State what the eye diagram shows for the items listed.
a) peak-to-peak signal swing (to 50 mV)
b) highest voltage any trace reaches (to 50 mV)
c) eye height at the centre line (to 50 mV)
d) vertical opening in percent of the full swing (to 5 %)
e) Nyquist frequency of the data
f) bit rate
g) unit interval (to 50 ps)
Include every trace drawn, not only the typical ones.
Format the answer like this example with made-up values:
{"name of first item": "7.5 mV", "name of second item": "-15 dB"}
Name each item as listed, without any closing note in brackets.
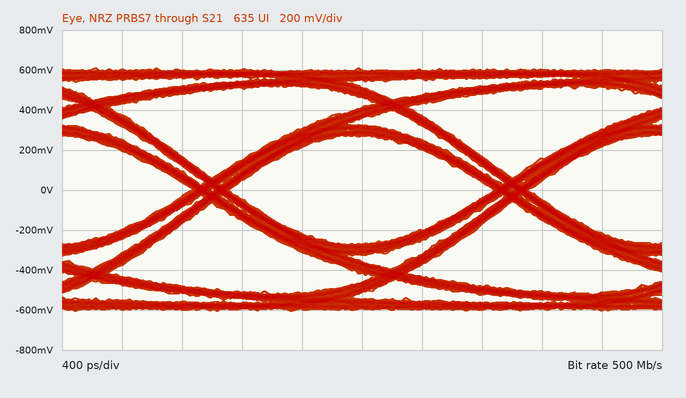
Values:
{"peak-to-peak signal swing": "1.20 V", "highest voltage any trace reaches": "600 mV", "eye height at the centre line": "550 mV", "vertical opening in percent of the full swing": "45 %", "Nyquist frequency of the data": "250 MHz", "bit rate": "500 Mb/s", "unit interval": "2.00 ns"}
